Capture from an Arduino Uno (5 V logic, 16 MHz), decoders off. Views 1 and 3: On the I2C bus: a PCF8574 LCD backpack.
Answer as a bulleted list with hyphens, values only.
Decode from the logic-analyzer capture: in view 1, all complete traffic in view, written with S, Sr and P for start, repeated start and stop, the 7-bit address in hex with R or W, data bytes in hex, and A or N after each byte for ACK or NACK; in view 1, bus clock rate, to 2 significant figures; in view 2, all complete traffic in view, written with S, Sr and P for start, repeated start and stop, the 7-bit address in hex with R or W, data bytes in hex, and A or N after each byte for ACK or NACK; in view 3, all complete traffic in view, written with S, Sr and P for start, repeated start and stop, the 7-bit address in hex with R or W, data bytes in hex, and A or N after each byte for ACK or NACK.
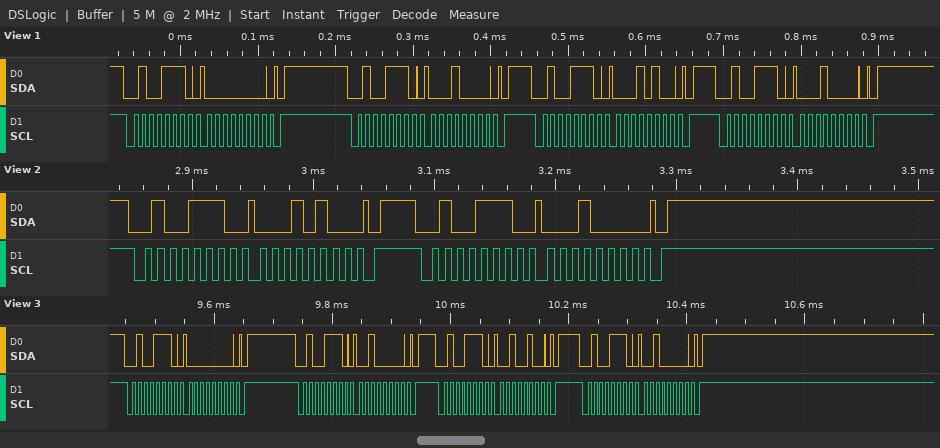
- S 27W A 00 A P S 27W A 10 A P S 27W A 14 A P S 27W A 10 A P
- 100 kHz
- S 27W A 14 A P S 27W A 10 A P
- S 27W A 00 A P S 27W A 20 A P S 27W A 24 A P S 27W A 20 A P
